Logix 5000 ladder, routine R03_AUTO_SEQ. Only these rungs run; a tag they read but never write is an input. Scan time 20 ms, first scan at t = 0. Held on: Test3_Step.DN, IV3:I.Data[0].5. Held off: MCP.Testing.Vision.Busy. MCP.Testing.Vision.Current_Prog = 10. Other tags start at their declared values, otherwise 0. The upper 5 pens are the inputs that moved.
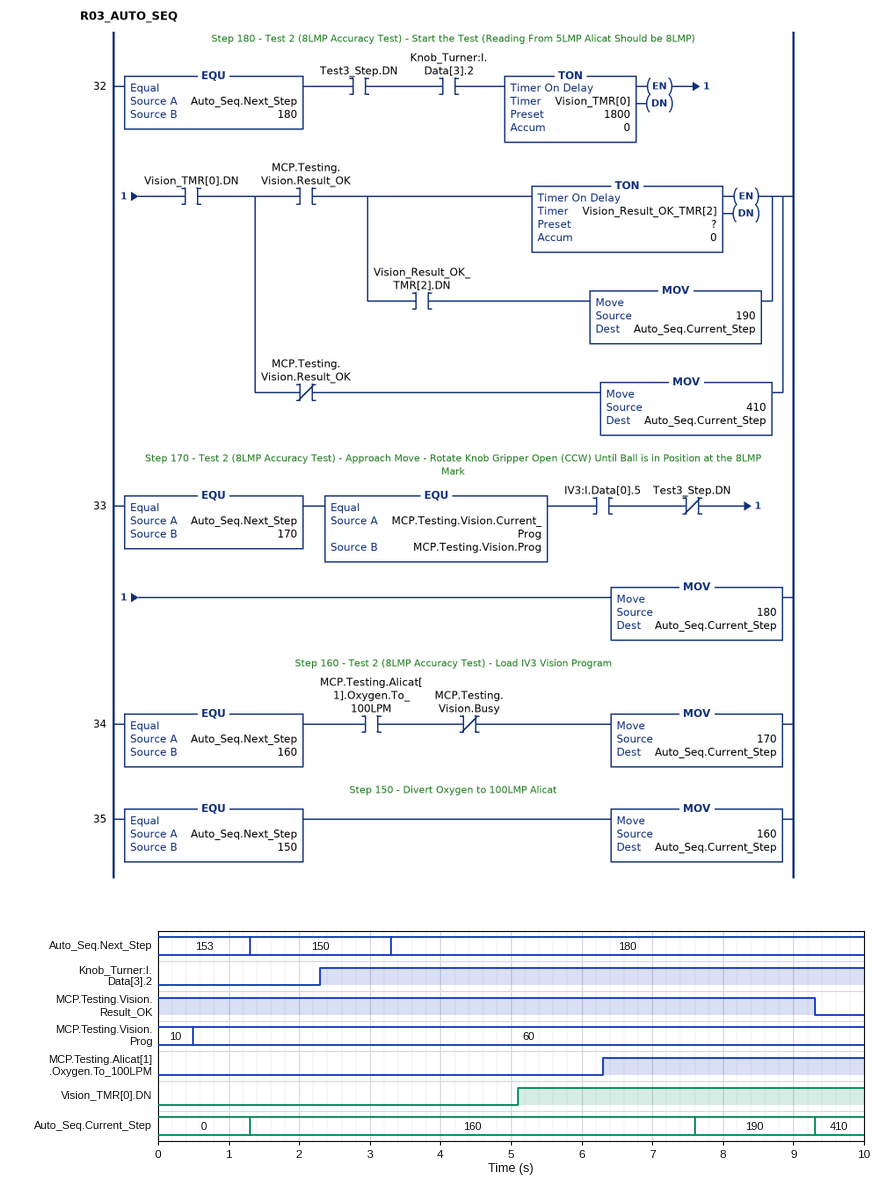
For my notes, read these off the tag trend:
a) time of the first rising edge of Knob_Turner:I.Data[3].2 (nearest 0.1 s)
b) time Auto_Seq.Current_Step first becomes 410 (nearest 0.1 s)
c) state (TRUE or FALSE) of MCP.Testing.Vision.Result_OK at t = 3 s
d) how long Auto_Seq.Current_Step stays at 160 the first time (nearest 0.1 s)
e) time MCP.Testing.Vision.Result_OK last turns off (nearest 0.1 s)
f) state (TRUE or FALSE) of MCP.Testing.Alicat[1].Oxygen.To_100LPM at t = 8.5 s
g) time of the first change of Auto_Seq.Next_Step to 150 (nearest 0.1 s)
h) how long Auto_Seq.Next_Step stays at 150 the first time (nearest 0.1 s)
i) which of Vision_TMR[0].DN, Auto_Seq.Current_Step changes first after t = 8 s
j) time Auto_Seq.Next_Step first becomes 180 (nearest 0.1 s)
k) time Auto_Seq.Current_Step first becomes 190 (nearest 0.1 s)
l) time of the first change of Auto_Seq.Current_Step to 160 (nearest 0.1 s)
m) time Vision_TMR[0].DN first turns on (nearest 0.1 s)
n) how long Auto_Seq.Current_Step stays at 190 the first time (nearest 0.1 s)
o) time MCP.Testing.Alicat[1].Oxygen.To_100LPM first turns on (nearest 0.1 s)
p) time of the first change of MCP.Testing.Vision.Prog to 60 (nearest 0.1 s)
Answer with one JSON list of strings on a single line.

["2.3 s", "9.3 s", "TRUE", "6.3 s", "9.3 s", "TRUE", "1.3 s", "2.0 s", "Auto_Seq.Current_Step", "3.3 s", "7.6 s", "1.3 s", "5.1 s", "1.7 s", "6.3 s", "0.5 s"]
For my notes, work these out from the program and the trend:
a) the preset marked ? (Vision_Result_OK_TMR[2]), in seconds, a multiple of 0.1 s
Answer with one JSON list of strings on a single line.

["2.5 s"]
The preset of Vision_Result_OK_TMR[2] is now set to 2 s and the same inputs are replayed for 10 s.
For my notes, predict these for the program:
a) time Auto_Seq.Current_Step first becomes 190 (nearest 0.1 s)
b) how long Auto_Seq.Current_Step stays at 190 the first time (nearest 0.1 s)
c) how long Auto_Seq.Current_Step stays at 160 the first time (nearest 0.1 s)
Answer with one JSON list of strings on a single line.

["7.1 s", "2.2 s", "5.8 s"]
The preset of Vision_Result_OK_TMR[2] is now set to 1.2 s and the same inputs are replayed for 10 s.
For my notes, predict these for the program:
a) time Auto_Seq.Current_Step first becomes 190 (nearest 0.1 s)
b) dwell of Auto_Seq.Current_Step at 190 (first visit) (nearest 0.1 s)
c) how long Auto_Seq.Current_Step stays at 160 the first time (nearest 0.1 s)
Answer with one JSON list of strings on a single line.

["6.3 s", "3.0 s", "5.0 s"]
